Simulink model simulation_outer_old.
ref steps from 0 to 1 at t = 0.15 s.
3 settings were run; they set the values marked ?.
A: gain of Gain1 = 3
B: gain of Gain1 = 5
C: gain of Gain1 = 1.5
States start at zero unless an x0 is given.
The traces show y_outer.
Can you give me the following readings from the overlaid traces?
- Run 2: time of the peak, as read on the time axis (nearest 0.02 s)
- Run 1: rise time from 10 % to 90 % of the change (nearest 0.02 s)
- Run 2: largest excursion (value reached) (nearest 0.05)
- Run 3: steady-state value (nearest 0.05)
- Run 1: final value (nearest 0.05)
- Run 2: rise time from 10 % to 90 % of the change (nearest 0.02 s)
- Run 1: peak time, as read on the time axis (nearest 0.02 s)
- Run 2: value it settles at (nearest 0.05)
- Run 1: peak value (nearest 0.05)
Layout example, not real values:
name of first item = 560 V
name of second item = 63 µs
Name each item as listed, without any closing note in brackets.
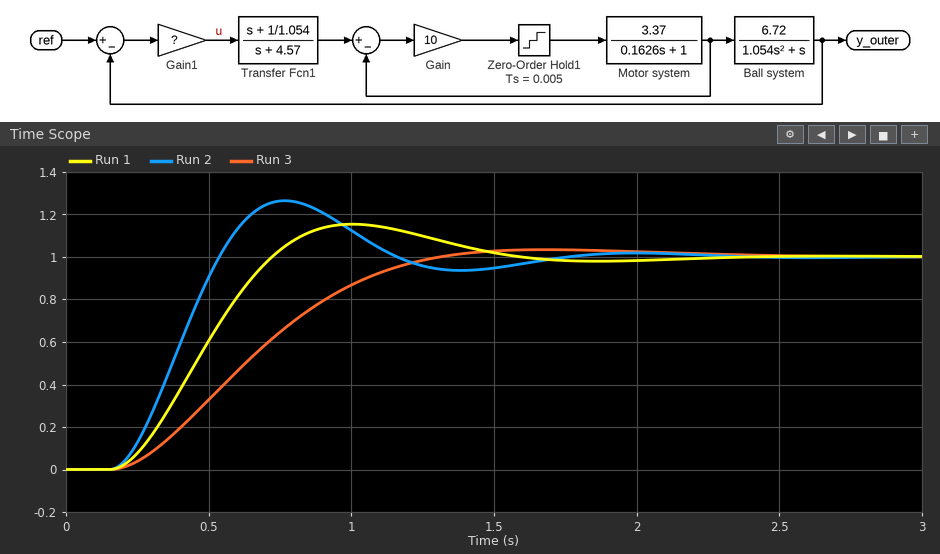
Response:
Run 2: time of the peak, as read on the time axis = 0.76 s
Run 1: rise time from 10 % to 90 % of the change = 0.38 s
Run 2: largest excursion (value reached) = 1.25
Run 3: steady-state value = 1.00
Run 1: final value = 1.00
Run 2: rise time from 10 % to 90 % of the change = 0.26 s
Run 1: peak time, as read on the time axis = 1.00 s
Run 2: value it settles at = 1.00
Run 1: peak value = 1.15
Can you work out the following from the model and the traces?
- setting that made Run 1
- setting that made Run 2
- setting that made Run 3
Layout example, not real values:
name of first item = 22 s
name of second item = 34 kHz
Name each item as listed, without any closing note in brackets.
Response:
setting that made Run 1 = A
setting that made Run 2 = B
setting that made Run 3 = C
